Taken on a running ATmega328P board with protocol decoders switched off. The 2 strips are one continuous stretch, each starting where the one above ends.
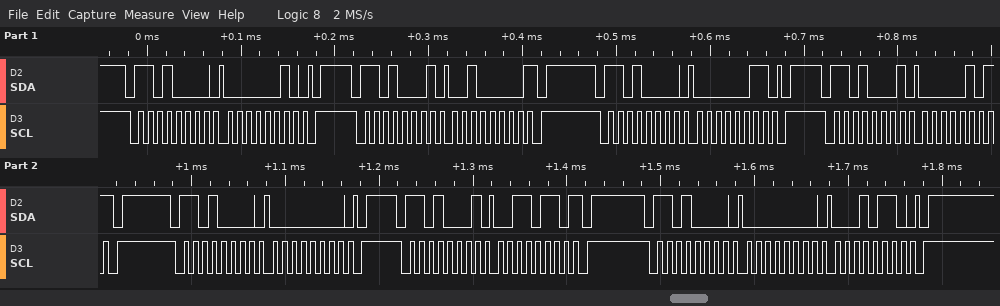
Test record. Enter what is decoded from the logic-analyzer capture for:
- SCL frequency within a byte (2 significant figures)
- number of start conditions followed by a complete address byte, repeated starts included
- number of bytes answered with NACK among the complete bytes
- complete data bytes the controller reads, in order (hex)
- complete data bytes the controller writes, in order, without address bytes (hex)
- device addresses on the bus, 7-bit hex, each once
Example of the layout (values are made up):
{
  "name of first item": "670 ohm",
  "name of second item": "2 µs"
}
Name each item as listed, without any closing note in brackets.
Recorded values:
{
  "SCL frequency within a byte": "100 kHz",
  "number of start conditions followed by a complete address byte, repeated starts included": "7",
  "number of bytes answered with NACK among the complete bytes": "3",
  "complete data bytes the controller reads, in order": "20 05 36",
  "complete data bytes the controller writes, in order, without address bytes": "02 03 00 00 16",
  "device addresses on the bus, 7-bit hex, each once": "0x68"
}
